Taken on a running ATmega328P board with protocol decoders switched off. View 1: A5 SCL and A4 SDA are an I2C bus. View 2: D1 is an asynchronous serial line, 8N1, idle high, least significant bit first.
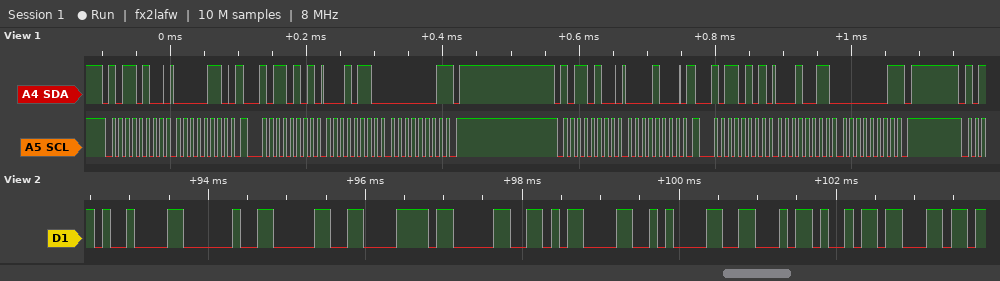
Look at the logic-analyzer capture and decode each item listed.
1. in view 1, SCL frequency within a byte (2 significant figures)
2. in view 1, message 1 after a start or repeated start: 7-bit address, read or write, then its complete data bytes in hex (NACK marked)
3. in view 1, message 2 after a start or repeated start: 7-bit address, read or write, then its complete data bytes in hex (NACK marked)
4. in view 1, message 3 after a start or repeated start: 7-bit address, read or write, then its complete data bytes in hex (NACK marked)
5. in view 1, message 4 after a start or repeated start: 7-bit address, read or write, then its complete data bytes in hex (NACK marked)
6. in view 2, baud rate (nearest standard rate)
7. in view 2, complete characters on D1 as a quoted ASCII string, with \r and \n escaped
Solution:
100 kHz
0x5A write: 06
0x5A read: 16 01 NACK
0x5A write: 08
0x5A read: 13 01 NACK
9600 baud
"\t 0x0\r\nFil"
